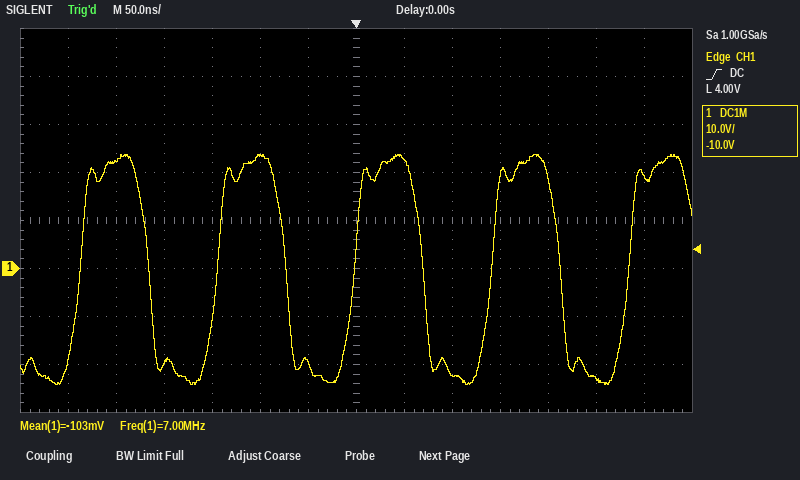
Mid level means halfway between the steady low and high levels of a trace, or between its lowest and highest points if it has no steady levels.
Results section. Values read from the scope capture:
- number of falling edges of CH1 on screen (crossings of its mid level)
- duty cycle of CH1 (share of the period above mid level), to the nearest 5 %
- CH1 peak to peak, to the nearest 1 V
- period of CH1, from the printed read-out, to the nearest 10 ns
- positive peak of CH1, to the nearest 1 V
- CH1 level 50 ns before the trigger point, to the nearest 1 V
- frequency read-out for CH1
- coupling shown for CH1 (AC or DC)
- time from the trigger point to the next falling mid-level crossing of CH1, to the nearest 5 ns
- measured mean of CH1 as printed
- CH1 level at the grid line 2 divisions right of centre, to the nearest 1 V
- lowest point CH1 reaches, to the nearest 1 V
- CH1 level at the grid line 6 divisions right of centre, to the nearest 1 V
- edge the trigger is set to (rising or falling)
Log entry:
4
50 %
48 V
140 ns
24 V
-20 V
7.00 MHz
DC
70 ns
-103 mV
-22 V
-24 V
19 V
rising
